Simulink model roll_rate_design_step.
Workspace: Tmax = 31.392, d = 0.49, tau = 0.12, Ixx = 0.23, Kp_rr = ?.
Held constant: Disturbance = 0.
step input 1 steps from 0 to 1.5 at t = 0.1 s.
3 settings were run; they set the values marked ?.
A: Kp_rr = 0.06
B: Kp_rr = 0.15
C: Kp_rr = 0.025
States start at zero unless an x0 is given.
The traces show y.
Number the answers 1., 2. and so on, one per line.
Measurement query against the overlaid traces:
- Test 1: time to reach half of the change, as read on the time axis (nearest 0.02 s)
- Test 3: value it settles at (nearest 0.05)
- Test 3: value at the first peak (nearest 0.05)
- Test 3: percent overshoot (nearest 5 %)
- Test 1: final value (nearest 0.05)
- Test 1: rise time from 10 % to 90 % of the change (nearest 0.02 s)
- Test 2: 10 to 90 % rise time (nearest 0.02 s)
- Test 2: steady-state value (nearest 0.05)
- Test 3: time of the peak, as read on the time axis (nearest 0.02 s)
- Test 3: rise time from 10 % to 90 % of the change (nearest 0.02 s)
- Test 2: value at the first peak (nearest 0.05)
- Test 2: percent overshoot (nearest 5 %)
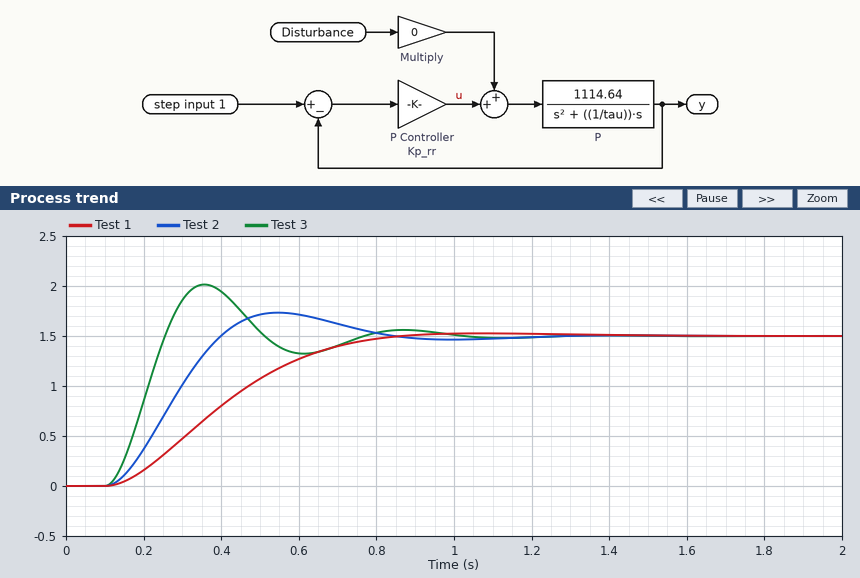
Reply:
1. 0.38 s
2. 1.50
3. 2.00
4. 35 %
5. 1.50
6. 0.46 s
7. 0.20 s
8. 1.50
9. 0.36 s
10. 0.10 s
11. 1.75
12. 15 %
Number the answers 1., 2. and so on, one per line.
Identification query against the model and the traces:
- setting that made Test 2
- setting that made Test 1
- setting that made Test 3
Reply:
1. A
2. C
3. B
